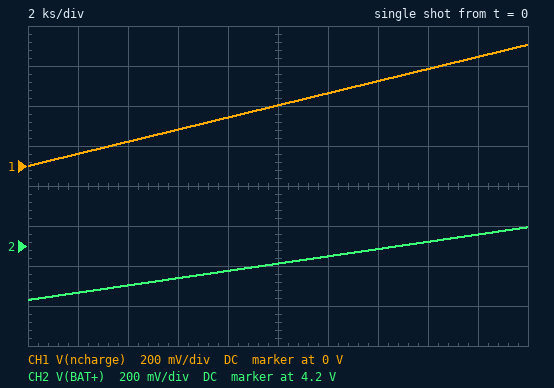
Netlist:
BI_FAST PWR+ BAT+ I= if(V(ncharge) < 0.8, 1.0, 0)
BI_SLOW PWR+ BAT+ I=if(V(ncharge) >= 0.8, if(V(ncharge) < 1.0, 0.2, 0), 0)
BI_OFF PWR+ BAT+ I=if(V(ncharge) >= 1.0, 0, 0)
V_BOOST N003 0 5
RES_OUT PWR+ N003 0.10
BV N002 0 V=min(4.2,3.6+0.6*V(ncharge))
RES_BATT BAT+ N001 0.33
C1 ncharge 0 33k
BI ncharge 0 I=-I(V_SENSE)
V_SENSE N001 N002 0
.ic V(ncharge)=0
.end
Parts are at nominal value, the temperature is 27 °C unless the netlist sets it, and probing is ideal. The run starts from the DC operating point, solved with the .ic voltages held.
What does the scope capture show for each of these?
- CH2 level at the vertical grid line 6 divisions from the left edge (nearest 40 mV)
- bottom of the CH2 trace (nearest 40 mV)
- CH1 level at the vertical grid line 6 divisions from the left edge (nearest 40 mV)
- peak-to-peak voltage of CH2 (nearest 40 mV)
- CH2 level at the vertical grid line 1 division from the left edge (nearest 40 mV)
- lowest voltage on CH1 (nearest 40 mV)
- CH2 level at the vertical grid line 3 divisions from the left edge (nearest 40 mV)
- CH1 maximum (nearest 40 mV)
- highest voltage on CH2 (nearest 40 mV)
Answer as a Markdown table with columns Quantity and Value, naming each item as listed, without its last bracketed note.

| Quantity | Value |
|---|---|
| CH2 level at the vertical grid line 6 divisions from the left edge | 4.16 V |
| bottom of the CH2 trace | 3.92 V |
| CH1 level at the vertical grid line 6 divisions from the left edge | 360 mV |
| peak-to-peak voltage of CH2 | 360 mV |
| CH2 level at the vertical grid line 1 division from the left edge | 3.96 V |
| lowest voltage on CH1 | 0 V |
| CH2 level at the vertical grid line 3 divisions from the left edge | 4.04 V |
| CH1 maximum | 600 mV |
| highest voltage on CH2 | 4.28 V |
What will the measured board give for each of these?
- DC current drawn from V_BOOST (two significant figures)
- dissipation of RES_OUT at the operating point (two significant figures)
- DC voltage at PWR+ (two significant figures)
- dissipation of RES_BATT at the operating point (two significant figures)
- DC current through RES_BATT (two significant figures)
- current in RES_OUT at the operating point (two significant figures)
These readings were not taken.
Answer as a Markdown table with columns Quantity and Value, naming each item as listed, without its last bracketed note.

| Quantity | Value |
|---|---|
| DC current drawn from V_BOOST | 1.0 A |
| dissipation of RES_OUT at the operating point | 100 mW |
| DC voltage at PWR+ | 4.9 V |
| dissipation of RES_BATT at the operating point | 330 mW |
| DC current through RES_BATT | 1.0 A |
| current in RES_OUT at the operating point | 1.0 A |
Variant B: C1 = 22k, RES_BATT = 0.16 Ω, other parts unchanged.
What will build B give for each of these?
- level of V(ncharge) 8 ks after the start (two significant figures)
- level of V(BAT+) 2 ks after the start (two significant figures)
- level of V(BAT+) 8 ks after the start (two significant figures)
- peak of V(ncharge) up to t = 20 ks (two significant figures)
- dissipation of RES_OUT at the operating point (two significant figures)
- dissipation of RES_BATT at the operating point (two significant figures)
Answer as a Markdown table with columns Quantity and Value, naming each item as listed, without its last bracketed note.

| Quantity | Value |
|---|---|
| level of V(ncharge) 8 ks after the start | 360 mV |
| level of V(BAT+) 2 ks after the start | 3.8 V |
| level of V(BAT+) 8 ks after the start | 4.0 V |
| peak of V(ncharge) up to t = 20 ks | 820 mV |
| dissipation of RES_OUT at the operating point | 100 mW |
| dissipation of RES_BATT at the operating point | 160 mW |
